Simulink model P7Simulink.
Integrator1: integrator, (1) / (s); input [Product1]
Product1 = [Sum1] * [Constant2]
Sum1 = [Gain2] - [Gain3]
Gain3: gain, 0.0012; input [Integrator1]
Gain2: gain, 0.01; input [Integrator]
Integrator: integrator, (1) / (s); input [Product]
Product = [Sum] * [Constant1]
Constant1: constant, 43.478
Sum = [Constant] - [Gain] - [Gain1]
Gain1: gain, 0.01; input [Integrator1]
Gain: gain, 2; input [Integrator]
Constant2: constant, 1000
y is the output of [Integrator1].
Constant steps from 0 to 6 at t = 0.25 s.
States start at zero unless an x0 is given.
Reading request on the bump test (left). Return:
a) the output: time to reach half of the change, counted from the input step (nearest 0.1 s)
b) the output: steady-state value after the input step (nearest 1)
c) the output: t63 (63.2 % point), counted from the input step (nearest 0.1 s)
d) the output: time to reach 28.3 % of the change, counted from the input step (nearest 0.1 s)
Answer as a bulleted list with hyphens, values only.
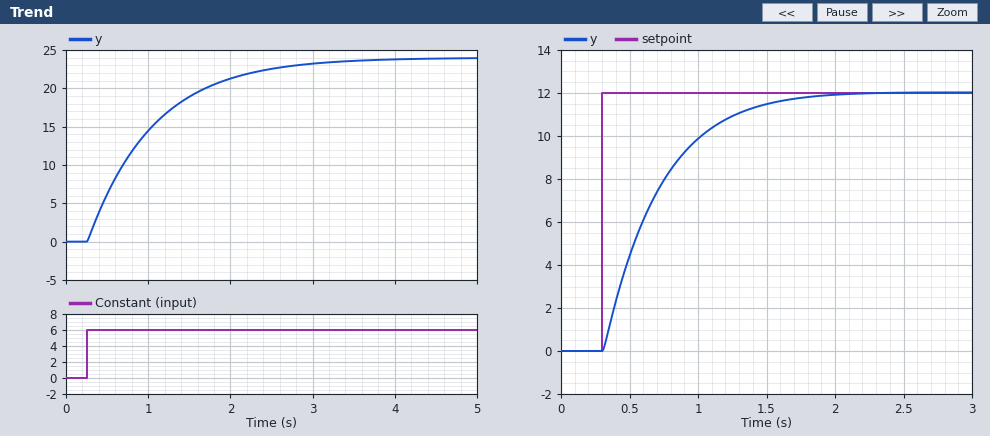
- 0.6 s
- 24
- 0.8 s
- 0.3 s
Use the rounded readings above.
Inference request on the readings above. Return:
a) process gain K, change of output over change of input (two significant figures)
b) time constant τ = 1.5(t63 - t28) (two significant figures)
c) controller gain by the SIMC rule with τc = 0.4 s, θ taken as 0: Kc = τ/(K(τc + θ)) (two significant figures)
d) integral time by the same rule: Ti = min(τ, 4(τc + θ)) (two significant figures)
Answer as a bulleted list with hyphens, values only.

- 4.0
- 0.75 s
- 0.47
- 0.75 s
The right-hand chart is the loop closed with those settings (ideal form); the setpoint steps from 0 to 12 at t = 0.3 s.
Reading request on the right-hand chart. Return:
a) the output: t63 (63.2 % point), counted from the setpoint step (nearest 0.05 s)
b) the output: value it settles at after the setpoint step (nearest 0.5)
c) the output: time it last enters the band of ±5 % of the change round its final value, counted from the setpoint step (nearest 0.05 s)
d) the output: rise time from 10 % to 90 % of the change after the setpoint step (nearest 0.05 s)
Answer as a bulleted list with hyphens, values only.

- 0.40 s
- 12.0
- 1.15 s
- 0.85 s
